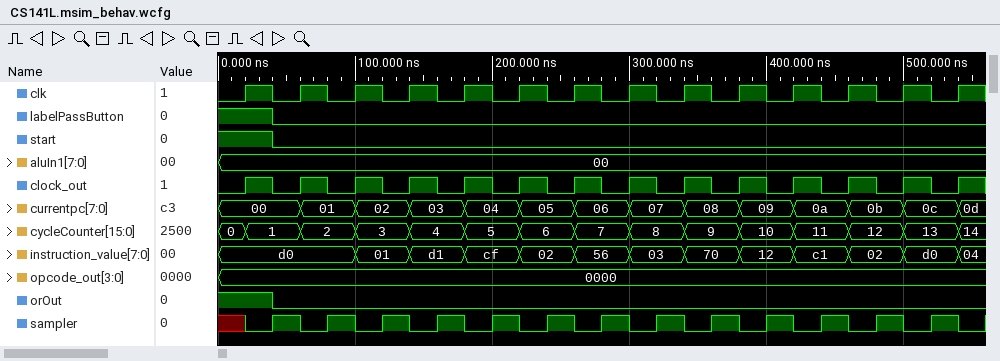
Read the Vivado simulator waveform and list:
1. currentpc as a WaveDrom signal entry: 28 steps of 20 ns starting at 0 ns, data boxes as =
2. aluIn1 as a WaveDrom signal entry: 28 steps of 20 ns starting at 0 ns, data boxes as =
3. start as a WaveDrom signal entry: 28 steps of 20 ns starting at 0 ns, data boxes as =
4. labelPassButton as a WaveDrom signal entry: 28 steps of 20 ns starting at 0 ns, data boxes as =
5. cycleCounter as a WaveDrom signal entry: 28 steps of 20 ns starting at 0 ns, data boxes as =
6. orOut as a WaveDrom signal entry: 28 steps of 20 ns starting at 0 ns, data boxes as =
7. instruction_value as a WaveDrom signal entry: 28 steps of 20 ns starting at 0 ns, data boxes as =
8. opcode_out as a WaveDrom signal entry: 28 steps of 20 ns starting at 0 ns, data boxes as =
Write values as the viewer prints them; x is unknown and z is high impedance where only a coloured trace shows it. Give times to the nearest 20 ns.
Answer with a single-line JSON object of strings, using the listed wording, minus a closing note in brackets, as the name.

{"currentpc as a WaveDrom signal entry: 28 steps of 20 ns starting at 0 ns, data boxes as =": "{name: 'currentpc', wave: '=..=.=.=.=.=.=.=.=.=.=.=.=.=', data: '00 01 02 03 04 05 06 07 08 09 0a 0b 0c 0d'}", "aluIn1 as a WaveDrom signal entry: 28 steps of 20 ns starting at 0 ns, data boxes as =": "{name: 'aluIn1', wave: '=...........................', data: '00'}", "start as a WaveDrom signal entry: 28 steps of 20 ns starting at 0 ns, data boxes as =": "{name: 'start', wave: '1.0.........................'}", "labelPassButton as a WaveDrom signal entry: 28 steps of 20 ns starting at 0 ns, data boxes as =": "{name: 'labelPassButton', wave: '1.0.........................'}", "cycleCounter as a WaveDrom signal entry: 28 steps of 20 ns starting at 0 ns, data boxes as =": "{name: 'cycleCounter', wave: '==.=.=.=.=.=.=.=.=.=.=.=.=.=', data: '0 1 2 3 4 5 6 7 8 9 10 11 12 13 14'}", "orOut as a WaveDrom signal entry: 28 steps of 20 ns starting at 0 ns, data boxes as =": "{name: 'orOut', wave: '1.0.........................'}", "instruction_value as a WaveDrom signal entry: 28 steps of 20 ns starting at 0 ns, data boxes as =": "{name: 'instruction_value', wave: '=....=.=.=.=.=.=.=.=.=.=.=.=', data: 'd0 01 d1 cf 02 56 03 70 12 c1 02 d0 04'}", "opcode_out as a WaveDrom signal entry: 28 steps of 20 ns starting at 0 ns, data boxes as =": "{name: 'opcode_out', wave: '=...........................', data: '0000'}"}
